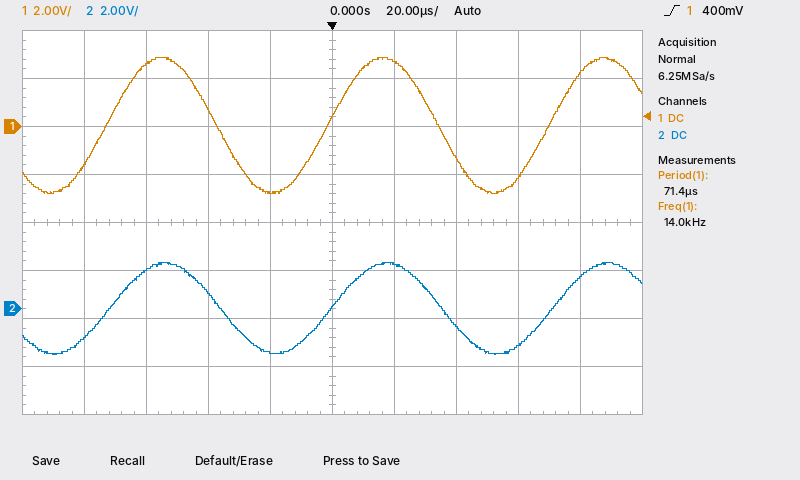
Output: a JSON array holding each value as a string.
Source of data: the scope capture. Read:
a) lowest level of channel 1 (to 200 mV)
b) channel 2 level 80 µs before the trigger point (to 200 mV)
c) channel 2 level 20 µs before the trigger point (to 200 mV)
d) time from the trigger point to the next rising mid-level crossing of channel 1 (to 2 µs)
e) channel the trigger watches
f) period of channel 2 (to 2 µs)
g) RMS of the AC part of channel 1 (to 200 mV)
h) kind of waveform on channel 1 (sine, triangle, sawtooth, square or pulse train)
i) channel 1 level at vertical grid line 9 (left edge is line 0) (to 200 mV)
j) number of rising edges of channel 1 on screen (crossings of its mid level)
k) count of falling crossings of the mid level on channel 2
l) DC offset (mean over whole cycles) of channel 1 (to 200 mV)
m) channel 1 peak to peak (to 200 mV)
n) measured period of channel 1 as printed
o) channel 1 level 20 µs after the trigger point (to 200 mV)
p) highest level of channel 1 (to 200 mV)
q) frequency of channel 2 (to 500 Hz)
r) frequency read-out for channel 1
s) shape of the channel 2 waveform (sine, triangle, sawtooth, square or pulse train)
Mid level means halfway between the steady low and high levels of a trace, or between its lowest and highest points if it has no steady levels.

["-2.8 V", "-1.2 V", "-1.8 V", "70 µs", "channel 1", "72 µs", "2.0 V", "sine", "2.2 V", "3", "2", "0.0 V", "5.6 V", "71.4 µs", "2.8 V", "2.8 V", "14.0 kHz", "14.0 kHz", "sine"]
